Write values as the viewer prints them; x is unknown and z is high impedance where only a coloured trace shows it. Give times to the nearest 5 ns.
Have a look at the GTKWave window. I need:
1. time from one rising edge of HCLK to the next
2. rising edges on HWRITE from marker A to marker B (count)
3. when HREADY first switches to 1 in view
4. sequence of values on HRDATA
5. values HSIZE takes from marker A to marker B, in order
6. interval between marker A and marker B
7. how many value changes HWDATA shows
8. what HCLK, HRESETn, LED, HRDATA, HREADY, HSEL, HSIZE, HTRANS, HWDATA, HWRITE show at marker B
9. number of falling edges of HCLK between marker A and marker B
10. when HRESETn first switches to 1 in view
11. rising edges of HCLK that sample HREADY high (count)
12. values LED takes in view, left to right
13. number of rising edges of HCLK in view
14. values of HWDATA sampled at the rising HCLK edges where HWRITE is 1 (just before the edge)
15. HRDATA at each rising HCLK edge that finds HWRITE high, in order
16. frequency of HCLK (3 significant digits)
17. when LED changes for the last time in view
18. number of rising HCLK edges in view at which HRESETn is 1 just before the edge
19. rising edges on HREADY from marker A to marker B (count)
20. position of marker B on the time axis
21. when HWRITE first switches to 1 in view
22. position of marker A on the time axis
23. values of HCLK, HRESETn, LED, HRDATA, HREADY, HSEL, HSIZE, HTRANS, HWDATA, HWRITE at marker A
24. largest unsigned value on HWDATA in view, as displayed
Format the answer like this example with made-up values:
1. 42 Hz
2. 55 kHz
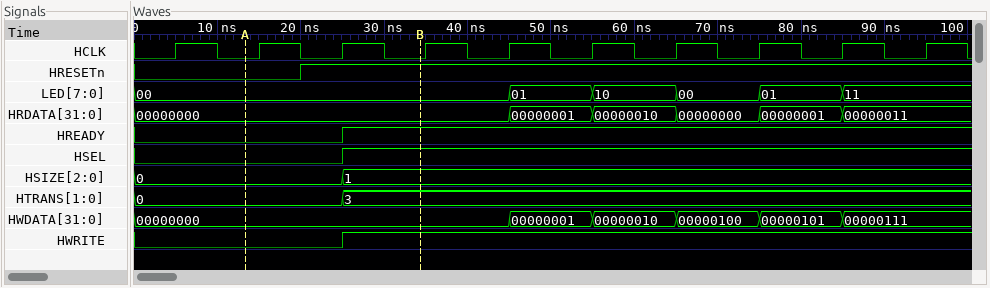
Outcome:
1. 10 ns
2. 1
3. 25 ns
4. 00000000, 00000001, 00000010, 00000000, 00000001, 00000011
5. 0, 1
6. 20 ns
7. 5
8. HCLK=0, HRESETn=1, LED=00, HRDATA=00000000, HREADY=1, HSEL=1, HSIZE=1, HTRANS=3, HWDATA=00000000, HWRITE=1
9. 2
10. 20 ns
11. 7
12. 00, 01, 10, 00, 01, 11
13. 10
14. 00000000, 00000000, 00000001, 00000010, 00000100, 00000101, 00000111
15. 00000000, 00000000, 00000001, 00000010, 00000000, 00000001, 00000011
16. 100 MHz
17. 85 ns
18. 8
19. 1
20. 35 ns
21. 25 ns
22. 15 ns
23. HCLK=0, HRESETn=0, LED=00, HRDATA=00000000, HREADY=0, HSEL=0, HSIZE=0, HTRANS=0, HWDATA=00000000, HWRITE=0
24. 00000111
